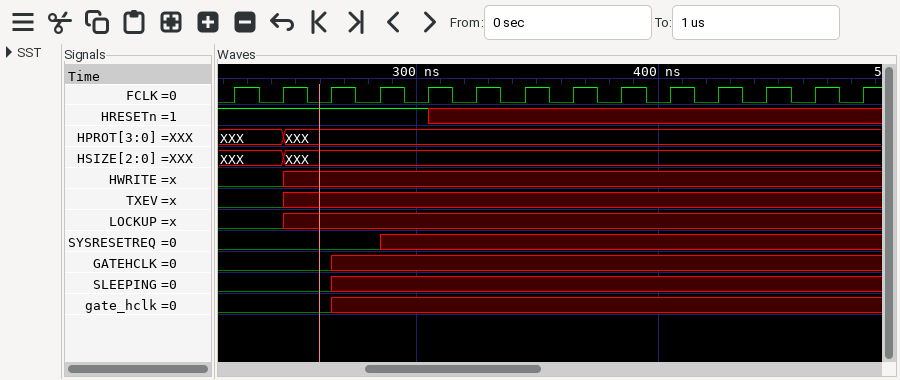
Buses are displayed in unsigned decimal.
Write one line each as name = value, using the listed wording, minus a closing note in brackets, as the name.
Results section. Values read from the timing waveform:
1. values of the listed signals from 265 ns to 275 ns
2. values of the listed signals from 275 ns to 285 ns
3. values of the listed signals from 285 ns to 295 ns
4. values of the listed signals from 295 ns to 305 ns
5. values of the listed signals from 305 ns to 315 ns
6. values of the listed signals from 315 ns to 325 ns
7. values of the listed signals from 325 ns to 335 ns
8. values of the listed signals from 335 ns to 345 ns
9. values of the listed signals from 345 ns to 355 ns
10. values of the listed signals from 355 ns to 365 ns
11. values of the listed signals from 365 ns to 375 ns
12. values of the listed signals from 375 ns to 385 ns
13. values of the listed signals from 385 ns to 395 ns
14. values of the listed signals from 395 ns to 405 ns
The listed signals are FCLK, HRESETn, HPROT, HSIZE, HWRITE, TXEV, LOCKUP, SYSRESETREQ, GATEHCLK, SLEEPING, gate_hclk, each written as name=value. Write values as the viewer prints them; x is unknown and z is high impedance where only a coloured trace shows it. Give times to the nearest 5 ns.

values of the listed signals from 265 ns to 275 ns = FCLK=1, HRESETn=1, HPROT=XXX, HSIZE=XXX, HWRITE=x, TXEV=x, LOCKUP=x, SYSRESETREQ=0, GATEHCLK=x, SLEEPING=x, gate_hclk=x
values of the listed signals from 275 ns to 285 ns = FCLK=0, HRESETn=1, HPROT=XXX, HSIZE=XXX, HWRITE=x, TXEV=x, LOCKUP=x, SYSRESETREQ=0, GATEHCLK=x, SLEEPING=x, gate_hclk=x
values of the listed signals from 285 ns to 295 ns = FCLK=1, HRESETn=1, HPROT=XXX, HSIZE=XXX, HWRITE=x, TXEV=x, LOCKUP=x, SYSRESETREQ=x, GATEHCLK=x, SLEEPING=x, gate_hclk=x
values of the listed signals from 295 ns to 305 ns = FCLK=0, HRESETn=1, HPROT=XXX, HSIZE=XXX, HWRITE=x, TXEV=x, LOCKUP=x, SYSRESETREQ=x, GATEHCLK=x, SLEEPING=x, gate_hclk=x
values of the listed signals from 305 ns to 315 ns = FCLK=1, HRESETn=x, HPROT=XXX, HSIZE=XXX, HWRITE=x, TXEV=x, LOCKUP=x, SYSRESETREQ=x, GATEHCLK=x, SLEEPING=x, gate_hclk=x
values of the listed signals from 315 ns to 325 ns = FCLK=0, HRESETn=x, HPROT=XXX, HSIZE=XXX, HWRITE=x, TXEV=x, LOCKUP=x, SYSRESETREQ=x, GATEHCLK=x, SLEEPING=x, gate_hclk=x
values of the listed signals from 325 ns to 335 ns = FCLK=1, HRESETn=x, HPROT=XXX, HSIZE=XXX, HWRITE=x, TXEV=x, LOCKUP=x, SYSRESETREQ=x, GATEHCLK=x, SLEEPING=x, gate_hclk=x
values of the listed signals from 335 ns to 345 ns = FCLK=0, HRESETn=x, HPROT=XXX, HSIZE=XXX, HWRITE=x, TXEV=x, LOCKUP=x, SYSRESETREQ=x, GATEHCLK=x, SLEEPING=x, gate_hclk=x
values of the listed signals from 345 ns to 355 ns = FCLK=1, HRESETn=x, HPROT=XXX, HSIZE=XXX, HWRITE=x, TXEV=x, LOCKUP=x, SYSRESETREQ=x, GATEHCLK=x, SLEEPING=x, gate_hclk=x
values of the listed signals from 355 ns to 365 ns = FCLK=0, HRESETn=x, HPROT=XXX, HSIZE=XXX, HWRITE=x, TXEV=x, LOCKUP=x, SYSRESETREQ=x, GATEHCLK=x, SLEEPING=x, gate_hclk=x
values of the listed signals from 365 ns to 375 ns = FCLK=1, HRESETn=x, HPROT=XXX, HSIZE=XXX, HWRITE=x, TXEV=x, LOCKUP=x, SYSRESETREQ=x, GATEHCLK=x, SLEEPING=x, gate_hclk=x
values of the listed signals from 375 ns to 385 ns = FCLK=0, HRESETn=x, HPROT=XXX, HSIZE=XXX, HWRITE=x, TXEV=x, LOCKUP=x, SYSRESETREQ=x, GATEHCLK=x, SLEEPING=x, gate_hclk=x
values of the listed signals from 385 ns to 395 ns = FCLK=1, HRESETn=x, HPROT=XXX, HSIZE=XXX, HWRITE=x, TXEV=x, LOCKUP=x, SYSRESETREQ=x, GATEHCLK=x, SLEEPING=x, gate_hclk=x
values of the listed signals from 395 ns to 405 ns = FCLK=0, HRESETn=x, HPROT=XXX, HSIZE=XXX, HWRITE=x, TXEV=x, LOCKUP=x, SYSRESETREQ=x, GATEHCLK=x, SLEEPING=x, gate_hclk=x
